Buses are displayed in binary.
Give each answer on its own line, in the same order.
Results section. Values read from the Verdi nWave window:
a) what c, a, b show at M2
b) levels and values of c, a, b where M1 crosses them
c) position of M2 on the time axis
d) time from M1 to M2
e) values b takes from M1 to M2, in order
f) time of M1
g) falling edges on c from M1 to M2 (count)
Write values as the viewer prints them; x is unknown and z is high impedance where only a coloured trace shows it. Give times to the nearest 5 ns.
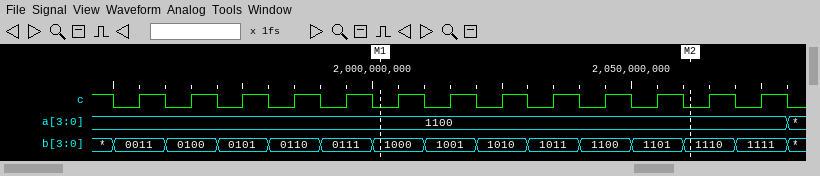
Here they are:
c=0, a=1100, b=1110
c=0, a=1100, b=1000
2060 ns
60 ns
1000, 1001, 1010, 1011, 1100, 1101, 1110
2000 ns
6
